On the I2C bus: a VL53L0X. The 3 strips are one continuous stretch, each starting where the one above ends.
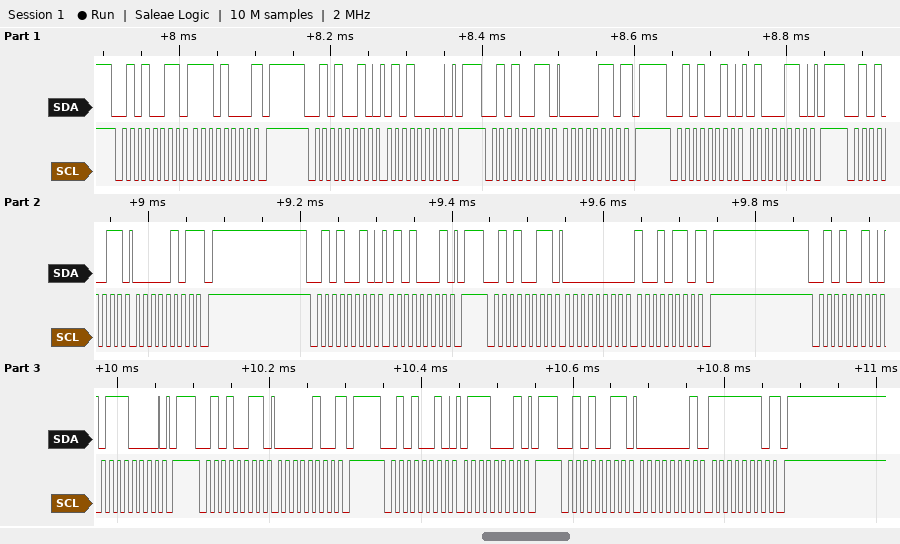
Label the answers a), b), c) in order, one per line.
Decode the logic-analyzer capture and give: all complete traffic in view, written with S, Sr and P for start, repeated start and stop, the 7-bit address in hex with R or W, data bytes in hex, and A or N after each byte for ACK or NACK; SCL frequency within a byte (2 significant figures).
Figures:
a) S 29R A E8 N P S 29W A 50 A P S 29R A 06 N P S 29W A 46 A P S 29R A 05 N P S 29W A 51 A P S 29R A 00 A 96 N P S 29W A 70 A P S 29R A 04 N P S 29W A 71 A P S 29R A 01 A FE N P
b) 100 kHz
